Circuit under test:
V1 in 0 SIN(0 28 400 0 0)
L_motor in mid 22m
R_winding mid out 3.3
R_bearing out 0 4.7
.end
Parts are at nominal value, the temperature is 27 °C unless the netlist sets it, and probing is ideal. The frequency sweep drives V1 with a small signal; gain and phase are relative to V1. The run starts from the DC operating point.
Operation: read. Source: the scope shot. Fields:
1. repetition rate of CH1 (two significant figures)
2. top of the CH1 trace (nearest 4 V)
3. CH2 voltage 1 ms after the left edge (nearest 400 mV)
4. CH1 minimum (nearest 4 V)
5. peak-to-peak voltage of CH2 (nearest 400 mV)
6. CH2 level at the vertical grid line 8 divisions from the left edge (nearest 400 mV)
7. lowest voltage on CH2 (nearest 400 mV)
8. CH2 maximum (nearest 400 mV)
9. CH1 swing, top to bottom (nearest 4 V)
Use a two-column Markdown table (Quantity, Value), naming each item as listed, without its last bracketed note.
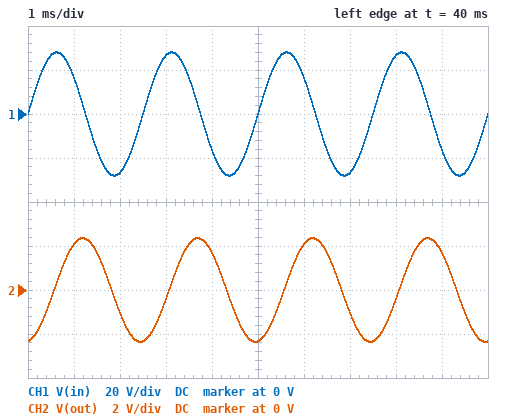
| Quantity | Value |
|---|---|
| repetition rate of CH1 | 400 Hz |
| top of the CH1 trace | 28 V |
| CH2 voltage 1 ms after the left edge | 2.0 V |
| CH1 minimum | -28 V |
| peak-to-peak voltage of CH2 | 4.8 V |
| CH2 level at the vertical grid line 8 divisions from the left edge | -400 mV |
| lowest voltage on CH2 | -2.4 V |
| CH2 maximum | 2.4 V |
| CH1 swing, top to bottom | 56 V |
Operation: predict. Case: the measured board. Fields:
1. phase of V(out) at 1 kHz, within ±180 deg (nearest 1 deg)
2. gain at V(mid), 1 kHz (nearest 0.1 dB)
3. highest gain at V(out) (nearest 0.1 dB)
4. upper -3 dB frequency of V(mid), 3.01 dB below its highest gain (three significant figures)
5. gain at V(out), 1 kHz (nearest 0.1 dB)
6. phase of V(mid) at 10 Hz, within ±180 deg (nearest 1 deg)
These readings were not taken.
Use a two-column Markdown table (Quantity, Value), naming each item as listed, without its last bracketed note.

| Quantity | Value |
|---|---|
| phase of V(out) at 1 kHz, within ±180 deg | -87 deg |
| gain at V(mid), 1 kHz | -24.8 dB |
| highest gain at V(out) | -4.6 dB |
| upper -3 dB frequency of V(mid), 3.01 dB below its highest gain | 57.9 Hz |
| gain at V(out), 1 kHz | -29.4 dB |
| phase of V(mid) at 10 Hz, within ±180 deg | -10 deg |
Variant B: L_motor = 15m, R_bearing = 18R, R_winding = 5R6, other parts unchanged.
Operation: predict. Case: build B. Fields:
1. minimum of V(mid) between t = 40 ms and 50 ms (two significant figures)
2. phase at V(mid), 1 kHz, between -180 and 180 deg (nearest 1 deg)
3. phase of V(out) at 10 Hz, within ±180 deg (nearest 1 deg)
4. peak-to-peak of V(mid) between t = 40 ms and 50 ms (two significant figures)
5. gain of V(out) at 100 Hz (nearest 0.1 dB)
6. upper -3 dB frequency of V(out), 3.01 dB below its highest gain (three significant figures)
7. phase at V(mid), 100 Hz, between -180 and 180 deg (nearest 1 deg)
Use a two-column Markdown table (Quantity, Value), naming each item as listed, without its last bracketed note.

| Quantity | Value |
|---|---|
| minimum of V(mid) between t = 40 ms and 50 ms | -15 V |
| phase at V(mid), 1 kHz, between -180 and 180 deg | -76 deg |
| phase of V(out) at 10 Hz, within ±180 deg | -2 deg |
| peak-to-peak of V(mid) between t = 40 ms and 50 ms | 30 V |
| gain of V(out) at 100 Hz | -3.0 dB |
| upper -3 dB frequency of V(out), 3.01 dB below its highest gain | 250 Hz |
| phase at V(mid), 100 Hz, between -180 and 180 deg | -22 deg |
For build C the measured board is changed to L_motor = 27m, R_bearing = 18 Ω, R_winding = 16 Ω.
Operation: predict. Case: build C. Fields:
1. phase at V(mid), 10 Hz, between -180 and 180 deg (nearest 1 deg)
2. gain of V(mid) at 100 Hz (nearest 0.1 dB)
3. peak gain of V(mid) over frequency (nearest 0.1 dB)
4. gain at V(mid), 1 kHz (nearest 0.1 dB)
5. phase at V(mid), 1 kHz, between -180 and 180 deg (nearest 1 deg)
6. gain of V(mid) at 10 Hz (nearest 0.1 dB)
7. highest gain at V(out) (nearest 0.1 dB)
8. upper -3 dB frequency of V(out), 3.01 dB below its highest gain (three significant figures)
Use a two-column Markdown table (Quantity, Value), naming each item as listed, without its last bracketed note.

| Quantity | Value |
|---|---|
| phase at V(mid), 10 Hz, between -180 and 180 deg | -3 deg |
| gain of V(mid) at 100 Hz | -1.0 dB |
| peak gain of V(mid) over frequency | 0 dB |
| gain at V(mid), 1 kHz | -14.1 dB |
| phase at V(mid), 1 kHz, between -180 and 180 deg | -79 deg |
| gain of V(mid) at 10 Hz | 0 dB |
| highest gain at V(out) | -5.5 dB |
| upper -3 dB frequency of V(out), 3.01 dB below its highest gain | 200 Hz |
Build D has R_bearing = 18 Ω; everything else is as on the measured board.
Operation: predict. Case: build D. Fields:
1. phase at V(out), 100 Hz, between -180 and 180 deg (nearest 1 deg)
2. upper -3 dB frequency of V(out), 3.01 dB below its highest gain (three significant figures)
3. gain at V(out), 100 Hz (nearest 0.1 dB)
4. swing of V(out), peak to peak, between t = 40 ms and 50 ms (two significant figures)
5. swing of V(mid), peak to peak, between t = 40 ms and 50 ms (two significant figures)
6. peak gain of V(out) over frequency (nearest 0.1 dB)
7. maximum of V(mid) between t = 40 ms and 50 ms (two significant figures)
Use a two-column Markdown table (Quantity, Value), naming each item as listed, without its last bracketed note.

| Quantity | Value |
|---|---|
| phase at V(out), 100 Hz, between -180 and 180 deg | -33 deg |
| upper -3 dB frequency of V(out), 3.01 dB below its highest gain | 154 Hz |
| gain at V(out), 100 Hz | -3.0 dB |
| swing of V(out), peak to peak, between t = 40 ms and 50 ms | 17 V |
| swing of V(mid), peak to peak, between t = 40 ms and 50 ms | 20 V |
| peak gain of V(out) over frequency | -1.5 dB |
| maximum of V(mid) between t = 40 ms and 50 ms | 10 V |
